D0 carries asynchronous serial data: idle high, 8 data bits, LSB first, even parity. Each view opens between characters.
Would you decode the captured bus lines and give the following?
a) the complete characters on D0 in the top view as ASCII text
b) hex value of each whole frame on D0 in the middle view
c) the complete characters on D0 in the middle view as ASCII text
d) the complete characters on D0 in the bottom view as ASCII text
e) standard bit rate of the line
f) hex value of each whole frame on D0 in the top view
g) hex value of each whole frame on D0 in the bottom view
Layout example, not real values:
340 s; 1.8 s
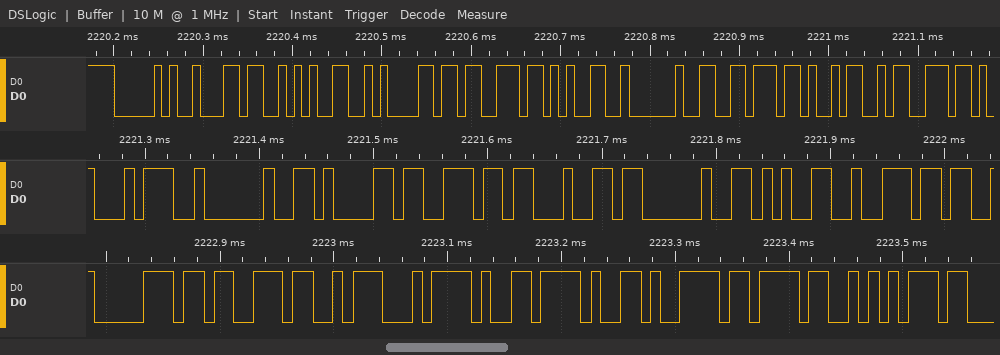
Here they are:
"Please vis"; 74, 20, 61, 6E, 64, 20, 65, 6E; "t and en"; "ps://you"; 115200 baud; 50, 6C, 65, 61, 73, 65, 20, 76, 69, 73; 70, 73, 3A, 2F, 2F, 79, 6F, 75
